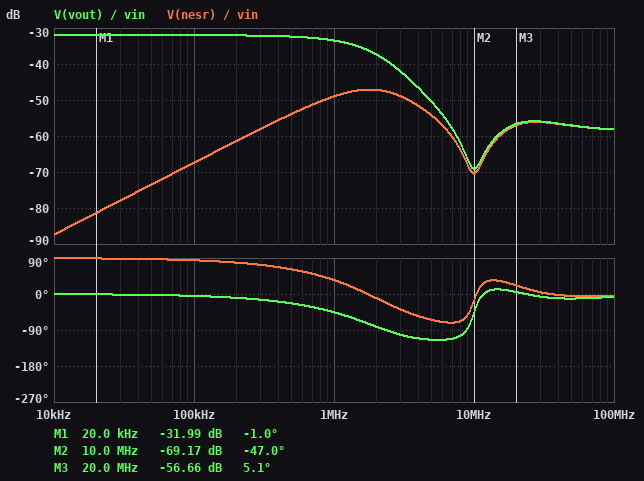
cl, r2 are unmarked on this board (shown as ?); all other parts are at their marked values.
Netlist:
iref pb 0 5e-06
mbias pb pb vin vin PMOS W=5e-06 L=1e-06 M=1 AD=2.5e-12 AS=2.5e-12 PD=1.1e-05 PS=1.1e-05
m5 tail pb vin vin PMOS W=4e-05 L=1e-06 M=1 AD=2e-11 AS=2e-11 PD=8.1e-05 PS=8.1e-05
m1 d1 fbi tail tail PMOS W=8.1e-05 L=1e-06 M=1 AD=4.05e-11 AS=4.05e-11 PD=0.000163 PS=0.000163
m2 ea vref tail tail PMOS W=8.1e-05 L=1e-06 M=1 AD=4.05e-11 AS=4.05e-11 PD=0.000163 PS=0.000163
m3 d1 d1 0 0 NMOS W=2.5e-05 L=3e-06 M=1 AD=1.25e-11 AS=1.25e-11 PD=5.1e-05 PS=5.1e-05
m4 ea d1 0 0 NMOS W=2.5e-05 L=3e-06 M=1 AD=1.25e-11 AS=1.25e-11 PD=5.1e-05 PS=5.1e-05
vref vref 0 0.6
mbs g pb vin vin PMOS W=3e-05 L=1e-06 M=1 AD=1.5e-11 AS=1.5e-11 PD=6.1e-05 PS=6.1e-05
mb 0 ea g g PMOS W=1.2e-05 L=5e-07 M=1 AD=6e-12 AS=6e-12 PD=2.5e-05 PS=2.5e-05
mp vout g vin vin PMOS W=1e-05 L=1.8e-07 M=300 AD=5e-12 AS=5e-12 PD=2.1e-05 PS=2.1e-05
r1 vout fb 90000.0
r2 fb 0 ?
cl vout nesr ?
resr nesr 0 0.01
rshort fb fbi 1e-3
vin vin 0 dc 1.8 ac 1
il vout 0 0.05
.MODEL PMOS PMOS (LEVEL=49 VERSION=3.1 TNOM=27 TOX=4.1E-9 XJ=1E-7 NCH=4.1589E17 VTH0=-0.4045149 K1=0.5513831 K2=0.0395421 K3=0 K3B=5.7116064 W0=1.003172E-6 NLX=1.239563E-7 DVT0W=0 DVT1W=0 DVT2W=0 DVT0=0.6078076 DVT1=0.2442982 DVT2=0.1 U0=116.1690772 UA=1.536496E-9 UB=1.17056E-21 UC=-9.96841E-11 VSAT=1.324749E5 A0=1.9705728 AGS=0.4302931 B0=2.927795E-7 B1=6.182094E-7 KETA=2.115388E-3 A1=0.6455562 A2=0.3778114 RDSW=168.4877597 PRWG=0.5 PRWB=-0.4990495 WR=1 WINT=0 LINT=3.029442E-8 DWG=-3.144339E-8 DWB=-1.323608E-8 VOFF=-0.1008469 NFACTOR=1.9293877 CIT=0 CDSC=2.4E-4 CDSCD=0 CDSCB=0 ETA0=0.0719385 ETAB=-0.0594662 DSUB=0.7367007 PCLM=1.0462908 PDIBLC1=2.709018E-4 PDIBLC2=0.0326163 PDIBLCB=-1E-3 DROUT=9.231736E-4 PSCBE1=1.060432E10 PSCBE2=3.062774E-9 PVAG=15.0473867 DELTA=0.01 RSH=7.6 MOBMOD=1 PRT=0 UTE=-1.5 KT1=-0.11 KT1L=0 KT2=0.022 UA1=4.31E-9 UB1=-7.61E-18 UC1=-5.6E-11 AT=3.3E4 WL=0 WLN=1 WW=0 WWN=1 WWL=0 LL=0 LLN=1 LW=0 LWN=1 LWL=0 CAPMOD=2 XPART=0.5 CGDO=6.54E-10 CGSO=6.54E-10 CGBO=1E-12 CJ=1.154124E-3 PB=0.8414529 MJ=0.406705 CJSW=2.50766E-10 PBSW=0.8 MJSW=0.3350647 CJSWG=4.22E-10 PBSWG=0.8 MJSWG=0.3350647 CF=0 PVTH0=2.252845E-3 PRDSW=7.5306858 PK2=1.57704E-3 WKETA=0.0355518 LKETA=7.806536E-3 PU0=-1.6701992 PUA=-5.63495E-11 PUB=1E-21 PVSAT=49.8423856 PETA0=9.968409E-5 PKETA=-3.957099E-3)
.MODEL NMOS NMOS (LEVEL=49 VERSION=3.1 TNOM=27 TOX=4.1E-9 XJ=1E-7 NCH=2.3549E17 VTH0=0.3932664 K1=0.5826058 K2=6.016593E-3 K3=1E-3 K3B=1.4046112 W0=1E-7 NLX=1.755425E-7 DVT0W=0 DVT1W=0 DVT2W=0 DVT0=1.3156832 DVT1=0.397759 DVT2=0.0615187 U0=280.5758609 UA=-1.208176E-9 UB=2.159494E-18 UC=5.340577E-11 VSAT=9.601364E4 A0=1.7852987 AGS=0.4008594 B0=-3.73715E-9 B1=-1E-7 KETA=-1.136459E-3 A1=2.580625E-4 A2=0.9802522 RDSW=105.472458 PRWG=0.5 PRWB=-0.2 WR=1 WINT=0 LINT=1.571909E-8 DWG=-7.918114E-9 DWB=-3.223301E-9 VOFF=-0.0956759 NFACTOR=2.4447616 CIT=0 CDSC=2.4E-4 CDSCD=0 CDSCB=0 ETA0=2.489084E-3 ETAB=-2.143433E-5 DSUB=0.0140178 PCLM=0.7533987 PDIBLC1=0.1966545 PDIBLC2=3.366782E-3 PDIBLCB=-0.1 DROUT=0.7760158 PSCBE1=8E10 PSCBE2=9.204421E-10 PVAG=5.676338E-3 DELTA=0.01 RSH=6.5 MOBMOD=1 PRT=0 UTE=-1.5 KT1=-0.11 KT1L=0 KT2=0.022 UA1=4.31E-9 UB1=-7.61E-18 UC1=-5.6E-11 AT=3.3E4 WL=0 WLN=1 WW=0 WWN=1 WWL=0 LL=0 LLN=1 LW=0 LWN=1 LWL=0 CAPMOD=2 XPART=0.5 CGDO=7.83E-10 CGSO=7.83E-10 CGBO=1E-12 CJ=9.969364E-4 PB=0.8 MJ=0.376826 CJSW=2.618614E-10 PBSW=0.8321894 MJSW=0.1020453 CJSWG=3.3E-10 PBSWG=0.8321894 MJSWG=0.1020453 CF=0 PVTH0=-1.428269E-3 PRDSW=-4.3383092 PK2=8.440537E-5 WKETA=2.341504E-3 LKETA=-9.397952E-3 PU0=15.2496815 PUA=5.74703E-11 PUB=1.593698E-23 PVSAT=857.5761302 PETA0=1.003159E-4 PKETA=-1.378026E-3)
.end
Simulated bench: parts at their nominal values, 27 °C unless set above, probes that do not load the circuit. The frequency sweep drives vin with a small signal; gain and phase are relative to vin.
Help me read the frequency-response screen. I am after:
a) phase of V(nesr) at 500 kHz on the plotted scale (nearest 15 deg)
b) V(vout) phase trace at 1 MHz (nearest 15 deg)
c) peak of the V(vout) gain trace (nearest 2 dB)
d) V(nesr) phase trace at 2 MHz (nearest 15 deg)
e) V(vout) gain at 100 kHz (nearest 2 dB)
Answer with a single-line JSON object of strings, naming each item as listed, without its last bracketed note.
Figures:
{"phase of V(nesr) at 500 kHz on the plotted scale": "60 deg", "V(vout) phase trace at 1 MHz": "-45 deg", "peak of the V(vout) gain trace": "-32 dB", "V(nesr) phase trace at 2 MHz": "-15 deg", "V(vout) gain at 100 kHz": "-32 dB"}
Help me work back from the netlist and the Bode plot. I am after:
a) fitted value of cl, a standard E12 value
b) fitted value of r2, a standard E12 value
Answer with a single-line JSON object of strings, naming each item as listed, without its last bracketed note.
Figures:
{"fitted value of cl, a standard E12 value": "2.7 µF", "fitted value of r2, a standard E12 value": "68 kΩ"}
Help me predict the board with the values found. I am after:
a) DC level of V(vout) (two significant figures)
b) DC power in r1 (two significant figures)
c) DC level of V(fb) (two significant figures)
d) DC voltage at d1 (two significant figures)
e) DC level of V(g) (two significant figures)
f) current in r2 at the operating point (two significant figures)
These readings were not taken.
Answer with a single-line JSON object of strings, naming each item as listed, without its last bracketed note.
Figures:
{"DC level of V(vout)": "1.4 V", "DC power in r1": "7.0 µW", "DC level of V(fb)": "600 mV", "DC voltage at d1": "560 mV", "DC level of V(g)": "1.0 V", "current in r2 at the operating point": "8.8 µA"}
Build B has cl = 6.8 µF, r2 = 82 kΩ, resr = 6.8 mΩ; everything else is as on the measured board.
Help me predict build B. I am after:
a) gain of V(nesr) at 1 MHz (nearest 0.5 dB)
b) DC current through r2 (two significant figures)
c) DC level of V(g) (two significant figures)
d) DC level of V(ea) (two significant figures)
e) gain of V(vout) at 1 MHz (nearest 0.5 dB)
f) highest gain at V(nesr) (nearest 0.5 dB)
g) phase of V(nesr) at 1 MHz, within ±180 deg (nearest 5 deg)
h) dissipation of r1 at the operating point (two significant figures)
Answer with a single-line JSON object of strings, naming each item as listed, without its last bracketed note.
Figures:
{"gain of V(nesr) at 1 MHz": "-52.0 dB", "DC current through r2": "7.3 µA", "DC level of V(g)": "1.0 V", "DC level of V(ea)": "390 mV", "gain of V(vout) at 1 MHz": "-41.0 dB", "highest gain at V(nesr)": "-51.5 dB", "phase of V(nesr) at 1 MHz, within ±180 deg": "10 deg", "dissipation of r1 at the operating point": "4.8 µW"}
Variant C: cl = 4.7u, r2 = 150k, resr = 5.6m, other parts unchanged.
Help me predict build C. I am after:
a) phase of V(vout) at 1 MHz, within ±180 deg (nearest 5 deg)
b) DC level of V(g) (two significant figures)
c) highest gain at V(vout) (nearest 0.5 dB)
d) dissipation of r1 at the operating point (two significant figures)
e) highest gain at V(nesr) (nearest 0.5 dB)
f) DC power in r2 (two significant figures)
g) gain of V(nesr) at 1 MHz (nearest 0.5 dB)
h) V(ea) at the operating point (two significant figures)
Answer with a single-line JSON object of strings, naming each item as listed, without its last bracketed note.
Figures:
{"phase of V(vout) at 1 MHz, within ±180 deg": "-55 deg", "DC level of V(g)": "1.0 V", "highest gain at V(vout)": "-35.5 dB", "dissipation of r1 at the operating point": "1.4 µW", "highest gain at V(nesr)": "-52.0 dB", "DC power in r2": "2.4 µW", "gain of V(nesr) at 1 MHz": "-53.5 dB", "V(ea) at the operating point": "400 mV"}
